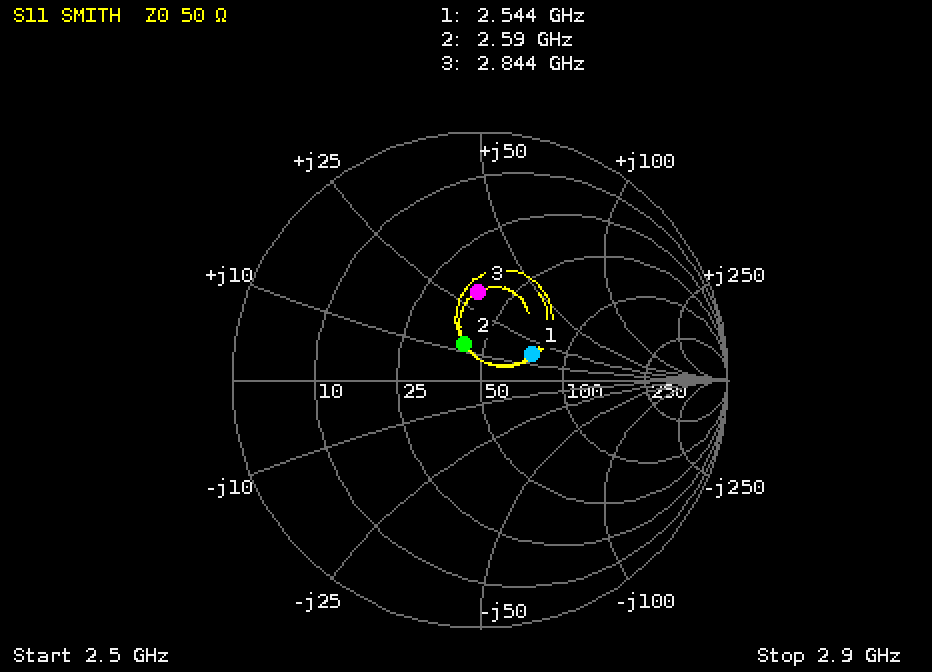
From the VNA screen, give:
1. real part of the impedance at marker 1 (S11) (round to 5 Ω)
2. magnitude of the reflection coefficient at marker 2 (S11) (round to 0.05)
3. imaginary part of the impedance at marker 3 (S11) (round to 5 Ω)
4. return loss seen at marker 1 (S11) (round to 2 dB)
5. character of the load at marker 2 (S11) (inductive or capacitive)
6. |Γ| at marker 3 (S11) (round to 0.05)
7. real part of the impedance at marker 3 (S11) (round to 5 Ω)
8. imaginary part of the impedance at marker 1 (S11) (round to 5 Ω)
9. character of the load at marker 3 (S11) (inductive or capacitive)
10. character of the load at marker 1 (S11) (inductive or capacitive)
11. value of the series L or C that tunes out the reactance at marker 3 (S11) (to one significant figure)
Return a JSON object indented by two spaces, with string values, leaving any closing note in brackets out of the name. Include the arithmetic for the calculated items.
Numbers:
{
  "real part of the impedance at marker 1 (S11)": "75 Ω",
  "magnitude of the reflection coefficient at marker 2 (S11)": "0.15",
  "imaginary part of the impedance at marker 3 (S11)": "+30 Ω",
  "return loss seen at marker 1 (S11)": "12 dB",
  "character of the load at marker 2 (S11)": "inductive",
  "|Γ| at marker 3 (S11)": "0.35",
  "real part of the impedance at marker 3 (S11)": "40 Ω",
  "imaginary part of the impedance at marker 1 (S11)": "+15 Ω",
  "character of the load at marker 3 (S11)": "inductive",
  "character of the load at marker 1 (S11)": "inductive",
  "value of the series L or C that tunes out the reactance at marker 3 (S11)": "C = 1/(2π × 2.844 GHz × 30 Ω) ≈ 2 pF"
}
